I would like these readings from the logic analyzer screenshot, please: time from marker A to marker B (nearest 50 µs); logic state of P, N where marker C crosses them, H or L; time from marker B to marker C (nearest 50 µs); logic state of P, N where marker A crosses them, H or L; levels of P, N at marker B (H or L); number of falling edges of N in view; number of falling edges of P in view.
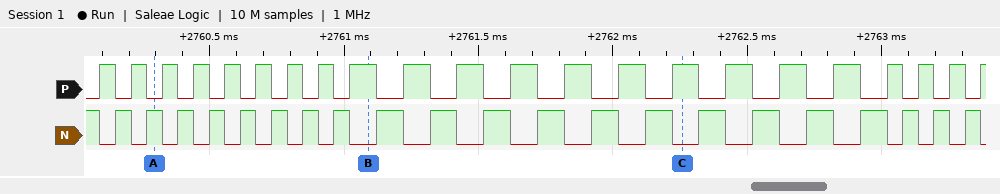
800 µs
P=H, N=L
1150 µs
P=L, N=H
P=H, N=L
22
21
